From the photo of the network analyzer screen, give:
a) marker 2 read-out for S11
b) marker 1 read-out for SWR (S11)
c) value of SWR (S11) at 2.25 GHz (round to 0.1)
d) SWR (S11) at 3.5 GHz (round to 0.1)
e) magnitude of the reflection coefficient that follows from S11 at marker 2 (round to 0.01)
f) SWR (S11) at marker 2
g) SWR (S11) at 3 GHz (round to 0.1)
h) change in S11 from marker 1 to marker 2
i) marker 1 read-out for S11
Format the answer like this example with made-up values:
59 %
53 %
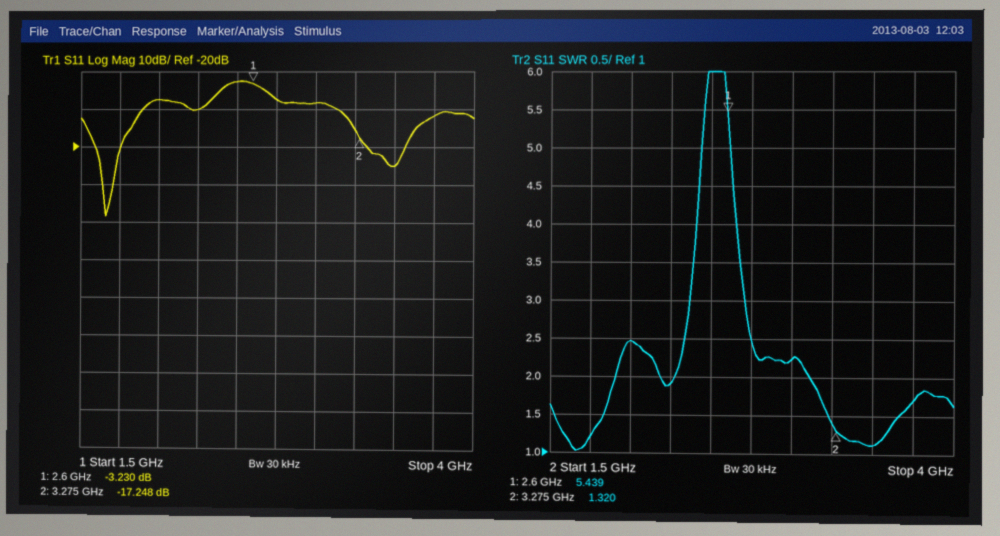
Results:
-17.248 dB
5.439
1.9
1.1
0.14
1.320
2.2
-14.018 dB
-3.230 dB
